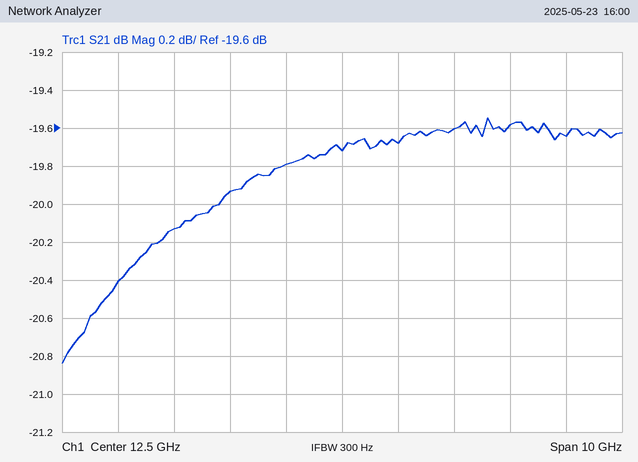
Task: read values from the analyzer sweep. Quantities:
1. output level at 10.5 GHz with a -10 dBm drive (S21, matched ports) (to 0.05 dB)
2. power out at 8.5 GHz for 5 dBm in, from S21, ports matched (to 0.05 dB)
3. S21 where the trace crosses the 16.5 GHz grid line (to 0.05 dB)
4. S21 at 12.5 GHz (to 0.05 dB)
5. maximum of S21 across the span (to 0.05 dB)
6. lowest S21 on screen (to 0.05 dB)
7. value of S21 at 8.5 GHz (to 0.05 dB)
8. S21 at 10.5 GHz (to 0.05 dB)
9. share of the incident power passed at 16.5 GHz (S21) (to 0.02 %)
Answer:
-29.95 dBm
-15.40 dBm
-19.65 dB
-19.70 dB
-19.55 dB
-20.85 dB
-20.40 dB
-19.95 dB
1.08 %
